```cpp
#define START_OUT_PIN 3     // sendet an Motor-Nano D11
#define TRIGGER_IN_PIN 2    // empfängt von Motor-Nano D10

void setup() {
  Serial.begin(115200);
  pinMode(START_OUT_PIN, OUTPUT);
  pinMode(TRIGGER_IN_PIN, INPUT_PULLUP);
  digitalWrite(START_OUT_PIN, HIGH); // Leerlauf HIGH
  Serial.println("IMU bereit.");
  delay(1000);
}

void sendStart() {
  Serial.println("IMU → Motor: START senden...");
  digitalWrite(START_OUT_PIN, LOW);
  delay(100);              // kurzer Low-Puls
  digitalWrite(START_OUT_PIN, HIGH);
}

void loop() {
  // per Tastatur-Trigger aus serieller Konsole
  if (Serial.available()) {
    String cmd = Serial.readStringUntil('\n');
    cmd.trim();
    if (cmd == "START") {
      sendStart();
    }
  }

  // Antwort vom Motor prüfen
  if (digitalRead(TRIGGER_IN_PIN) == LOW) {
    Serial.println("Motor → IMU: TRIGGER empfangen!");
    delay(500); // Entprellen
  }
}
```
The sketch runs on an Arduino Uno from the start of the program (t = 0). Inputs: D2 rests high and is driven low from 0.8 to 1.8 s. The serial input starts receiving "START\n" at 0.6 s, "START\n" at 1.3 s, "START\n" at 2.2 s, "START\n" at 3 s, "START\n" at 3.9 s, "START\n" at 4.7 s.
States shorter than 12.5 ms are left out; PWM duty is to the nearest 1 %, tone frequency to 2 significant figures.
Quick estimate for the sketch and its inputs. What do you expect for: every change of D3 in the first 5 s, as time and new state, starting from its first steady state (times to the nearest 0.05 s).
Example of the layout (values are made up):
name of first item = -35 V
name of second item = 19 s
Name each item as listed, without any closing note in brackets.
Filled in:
every change of D3 in the first 5 s, as time and new state, starting from its first steady state = 0 s high; 1 s low; 1.1 s high; 1.6 s low; 1.7 s high; 2.2 s low; 2.3 s high; 3 s low; 3.1 s high; 3.9 s low; 4 s high; 4.7 s low; 4.8 s high
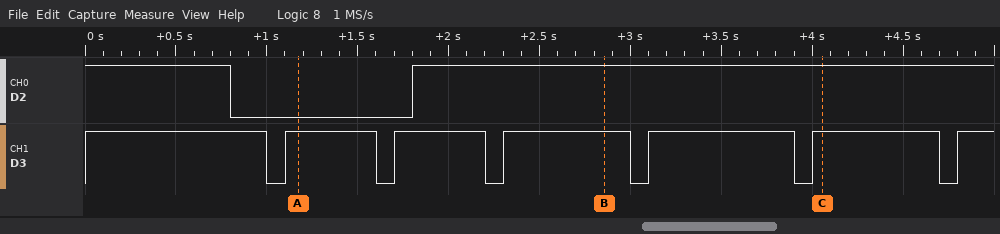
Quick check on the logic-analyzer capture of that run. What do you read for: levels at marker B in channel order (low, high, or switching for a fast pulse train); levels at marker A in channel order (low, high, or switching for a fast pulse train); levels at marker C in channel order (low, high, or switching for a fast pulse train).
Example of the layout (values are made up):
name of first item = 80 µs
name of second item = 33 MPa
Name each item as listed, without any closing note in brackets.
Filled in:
levels at marker B in channel order = D2 high, D3 high
levels at marker A in channel order = D2 low, D3 high
levels at marker C in channel order = D2 high, D3 high
